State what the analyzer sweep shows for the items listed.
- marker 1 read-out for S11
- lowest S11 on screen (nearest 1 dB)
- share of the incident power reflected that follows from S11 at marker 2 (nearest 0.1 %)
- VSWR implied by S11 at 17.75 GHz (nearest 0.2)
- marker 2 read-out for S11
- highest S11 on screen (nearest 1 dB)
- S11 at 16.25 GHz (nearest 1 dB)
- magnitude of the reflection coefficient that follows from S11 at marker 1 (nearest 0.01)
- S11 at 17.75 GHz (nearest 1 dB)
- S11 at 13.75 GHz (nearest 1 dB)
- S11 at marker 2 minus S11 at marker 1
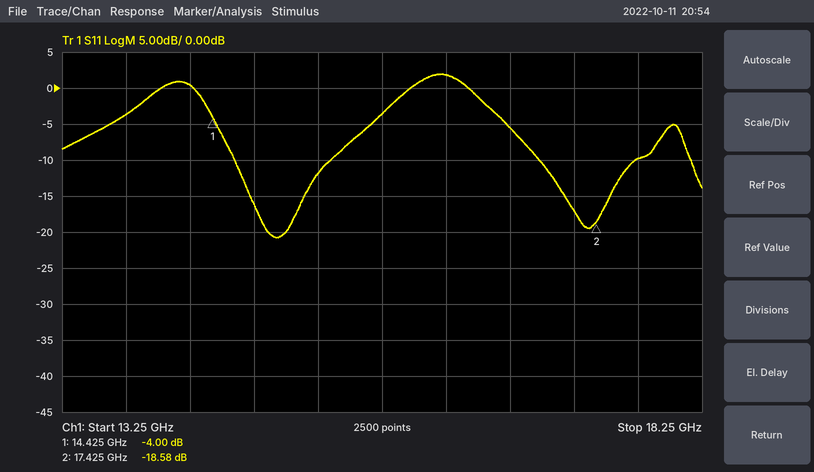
-4.00 dB
-21 dB
1.4 %
2.0
-18.58 dB
2 dB
2 dB
0.63
-10 dB
-4 dB
-14.58 dB
